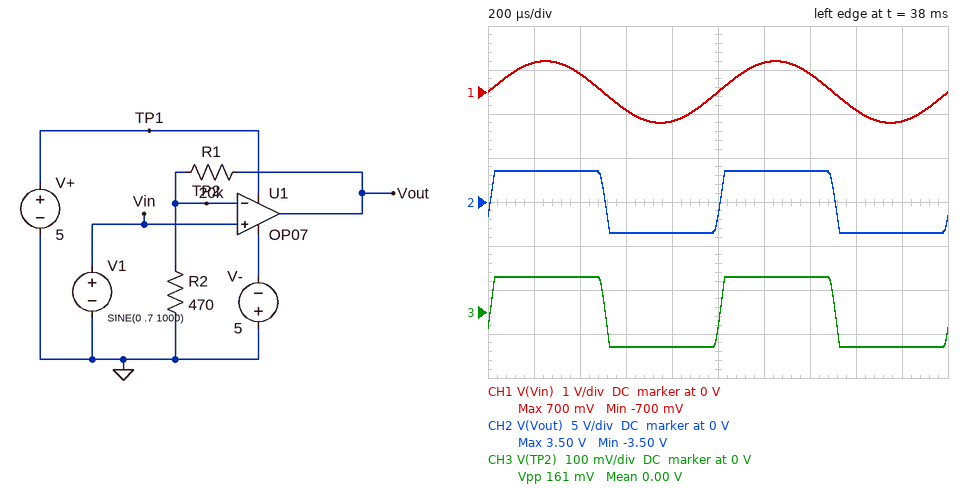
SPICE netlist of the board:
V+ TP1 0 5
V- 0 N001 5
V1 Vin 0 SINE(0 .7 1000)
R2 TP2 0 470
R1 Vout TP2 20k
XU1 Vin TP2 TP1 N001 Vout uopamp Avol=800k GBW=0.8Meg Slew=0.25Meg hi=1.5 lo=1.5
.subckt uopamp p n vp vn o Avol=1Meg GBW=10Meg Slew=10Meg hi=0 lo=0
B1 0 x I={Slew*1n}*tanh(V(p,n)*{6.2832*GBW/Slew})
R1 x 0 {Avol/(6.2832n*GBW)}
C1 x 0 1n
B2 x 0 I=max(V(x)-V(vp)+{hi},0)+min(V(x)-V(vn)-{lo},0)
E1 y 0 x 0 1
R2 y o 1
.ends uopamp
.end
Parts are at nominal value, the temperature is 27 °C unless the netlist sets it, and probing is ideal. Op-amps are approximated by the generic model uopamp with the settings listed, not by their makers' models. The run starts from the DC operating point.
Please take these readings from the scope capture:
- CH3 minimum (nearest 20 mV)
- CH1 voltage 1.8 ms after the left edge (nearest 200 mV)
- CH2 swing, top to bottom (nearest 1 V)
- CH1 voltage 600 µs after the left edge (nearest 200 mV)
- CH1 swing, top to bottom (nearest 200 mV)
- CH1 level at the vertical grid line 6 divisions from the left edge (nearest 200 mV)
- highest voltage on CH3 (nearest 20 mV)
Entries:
-80 mV
-600 mV
7 V
-400 mV
1.4 V
600 mV
80 mV
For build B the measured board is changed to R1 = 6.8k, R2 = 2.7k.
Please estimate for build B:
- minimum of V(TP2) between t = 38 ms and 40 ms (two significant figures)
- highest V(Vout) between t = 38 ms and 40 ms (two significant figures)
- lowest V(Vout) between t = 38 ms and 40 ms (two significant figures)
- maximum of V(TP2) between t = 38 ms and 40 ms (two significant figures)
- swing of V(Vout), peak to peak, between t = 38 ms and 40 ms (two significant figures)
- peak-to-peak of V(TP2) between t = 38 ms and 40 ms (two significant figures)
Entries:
-700 mV
2.5 V
-2.5 V
700 mV
4.9 V
1.4 V
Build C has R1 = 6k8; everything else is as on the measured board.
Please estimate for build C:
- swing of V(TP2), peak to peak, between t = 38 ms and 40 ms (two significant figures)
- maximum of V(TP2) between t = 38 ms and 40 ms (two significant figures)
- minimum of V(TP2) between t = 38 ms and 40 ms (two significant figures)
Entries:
450 mV
230 mV
-230 mV
